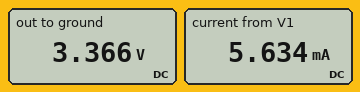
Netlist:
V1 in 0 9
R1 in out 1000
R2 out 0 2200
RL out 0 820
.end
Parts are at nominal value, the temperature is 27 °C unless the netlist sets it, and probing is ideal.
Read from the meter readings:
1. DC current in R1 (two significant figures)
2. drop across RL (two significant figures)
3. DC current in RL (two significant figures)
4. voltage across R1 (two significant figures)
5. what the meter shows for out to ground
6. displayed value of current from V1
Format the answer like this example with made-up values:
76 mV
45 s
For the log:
5.6 mA
3.4 V
4.1 mA
5.6 V
3.366 V
5.634 mA
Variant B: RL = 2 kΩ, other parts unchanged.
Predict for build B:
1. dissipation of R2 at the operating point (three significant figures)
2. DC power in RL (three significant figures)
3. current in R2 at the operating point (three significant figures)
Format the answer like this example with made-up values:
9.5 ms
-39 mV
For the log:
9.64 mW
10.6 mW
2.09 mA
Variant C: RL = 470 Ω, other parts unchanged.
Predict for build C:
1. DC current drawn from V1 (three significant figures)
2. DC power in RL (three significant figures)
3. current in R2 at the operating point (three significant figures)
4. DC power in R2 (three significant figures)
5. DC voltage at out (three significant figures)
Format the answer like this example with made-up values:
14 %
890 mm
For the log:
6.49 mA
13.4 mW
1.14 mA
2.87 mW
2.51 V
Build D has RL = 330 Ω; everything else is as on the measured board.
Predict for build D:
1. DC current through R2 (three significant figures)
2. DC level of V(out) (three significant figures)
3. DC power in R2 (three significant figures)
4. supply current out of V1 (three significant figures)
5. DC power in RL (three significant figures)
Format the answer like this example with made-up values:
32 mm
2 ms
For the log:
912 µA
2.01 V
1.83 mW
6.99 mA
12.2 mW
